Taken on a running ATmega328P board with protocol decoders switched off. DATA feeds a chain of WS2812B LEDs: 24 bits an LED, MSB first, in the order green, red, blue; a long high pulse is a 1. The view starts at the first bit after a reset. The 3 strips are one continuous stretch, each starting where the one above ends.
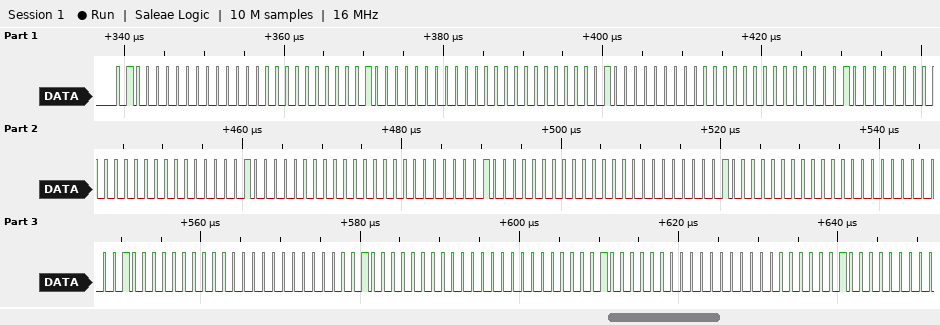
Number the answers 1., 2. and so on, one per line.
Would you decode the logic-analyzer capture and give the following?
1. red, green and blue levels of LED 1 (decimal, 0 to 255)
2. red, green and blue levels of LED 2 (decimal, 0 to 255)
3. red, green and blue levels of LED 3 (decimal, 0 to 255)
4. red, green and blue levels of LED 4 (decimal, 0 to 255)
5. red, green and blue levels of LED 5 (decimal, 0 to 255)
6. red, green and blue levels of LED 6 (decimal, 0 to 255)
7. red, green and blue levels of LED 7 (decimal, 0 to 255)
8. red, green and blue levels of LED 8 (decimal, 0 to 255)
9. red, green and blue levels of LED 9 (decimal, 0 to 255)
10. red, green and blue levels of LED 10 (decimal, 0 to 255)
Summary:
1. 0, 64, 0
2. 0, 64, 0
3. 0, 64, 0
4. 0, 64, 0
5. 0, 64, 0
6. 0, 64, 0
7. 0, 64, 0
8. 0, 64, 0
9. 0, 64, 0
10. 0, 64, 0
